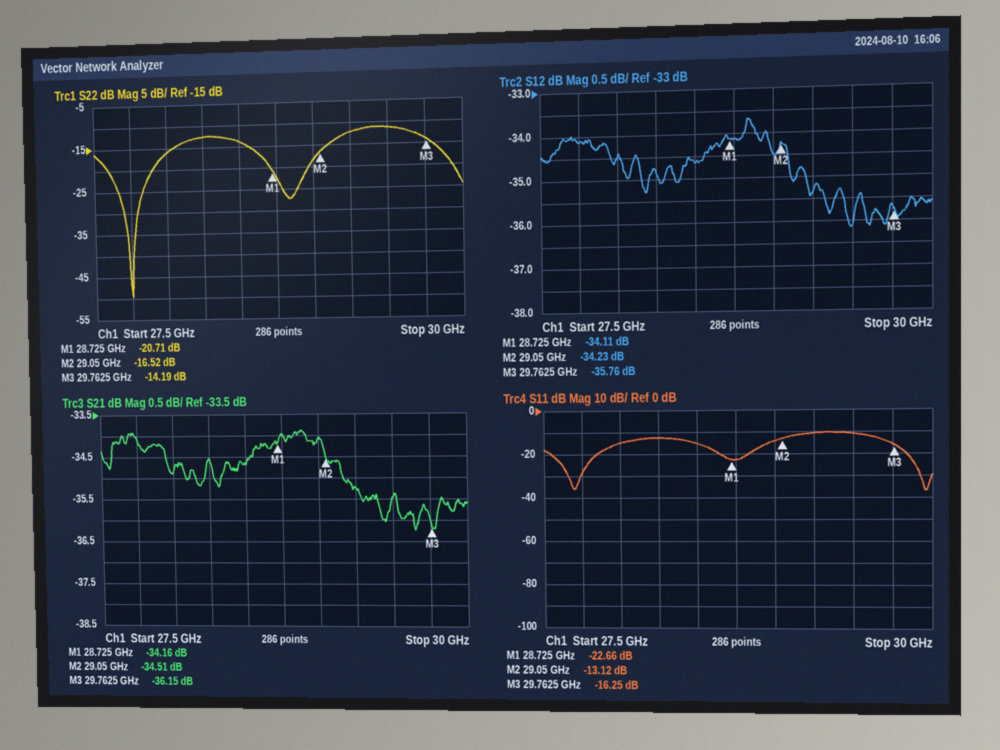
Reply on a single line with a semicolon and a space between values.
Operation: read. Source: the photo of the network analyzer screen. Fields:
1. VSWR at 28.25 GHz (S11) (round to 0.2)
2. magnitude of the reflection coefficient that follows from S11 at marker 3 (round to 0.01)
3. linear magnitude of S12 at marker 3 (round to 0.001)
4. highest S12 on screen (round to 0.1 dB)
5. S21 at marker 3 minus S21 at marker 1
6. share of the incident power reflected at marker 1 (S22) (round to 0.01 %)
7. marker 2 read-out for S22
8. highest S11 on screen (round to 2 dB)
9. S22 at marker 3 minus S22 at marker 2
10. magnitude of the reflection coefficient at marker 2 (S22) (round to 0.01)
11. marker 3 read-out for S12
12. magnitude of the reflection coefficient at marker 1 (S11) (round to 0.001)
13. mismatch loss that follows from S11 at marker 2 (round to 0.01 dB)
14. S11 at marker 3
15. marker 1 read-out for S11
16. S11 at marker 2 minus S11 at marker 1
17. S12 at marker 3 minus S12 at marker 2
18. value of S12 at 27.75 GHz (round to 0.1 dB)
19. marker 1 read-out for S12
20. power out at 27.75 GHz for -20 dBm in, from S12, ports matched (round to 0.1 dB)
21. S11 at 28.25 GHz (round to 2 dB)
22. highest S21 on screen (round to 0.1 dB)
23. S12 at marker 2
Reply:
1.6; 0.15; 0.016; -33.7 dB; -1.99 dB; 0.85 %; -16.52 dB; -10 dB; 2.33 dB; 0.15; -35.76 dB; 0.074; 0.22 dB; -16.25 dB; -22.66 dB; 9.54 dB; -1.53 dB; -34.1 dB; -34.11 dB; -54.1 dBm; -12 dB; -33.9 dB; -34.23 dB
